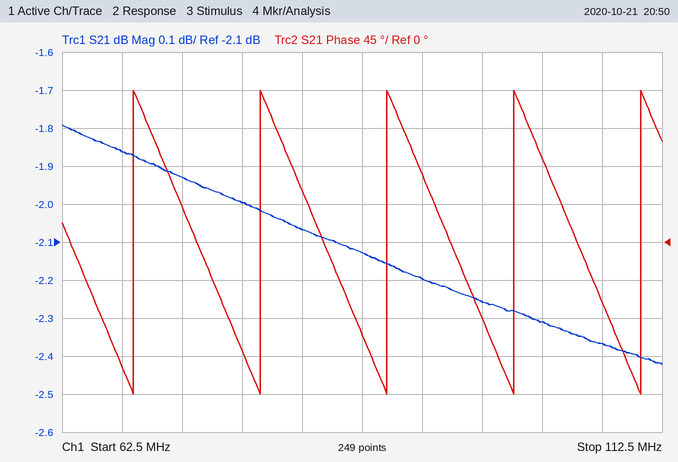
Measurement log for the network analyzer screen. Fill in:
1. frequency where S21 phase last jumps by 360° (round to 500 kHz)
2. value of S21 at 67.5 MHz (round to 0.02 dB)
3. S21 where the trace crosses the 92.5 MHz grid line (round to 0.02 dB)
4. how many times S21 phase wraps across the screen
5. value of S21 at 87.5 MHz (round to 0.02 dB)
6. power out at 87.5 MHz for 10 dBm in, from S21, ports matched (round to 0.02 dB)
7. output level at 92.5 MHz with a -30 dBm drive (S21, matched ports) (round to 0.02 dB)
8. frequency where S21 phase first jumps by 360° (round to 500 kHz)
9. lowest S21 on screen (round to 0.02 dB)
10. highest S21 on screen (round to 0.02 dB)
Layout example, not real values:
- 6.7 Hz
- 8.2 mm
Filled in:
- 110.5 MHz
- -1.86 dB
- -2.20 dB
- 5
- -2.12 dB
- 7.88 dBm
- -32.20 dBm
- 68.5 MHz
- -2.42 dB
- -1.80 dB
